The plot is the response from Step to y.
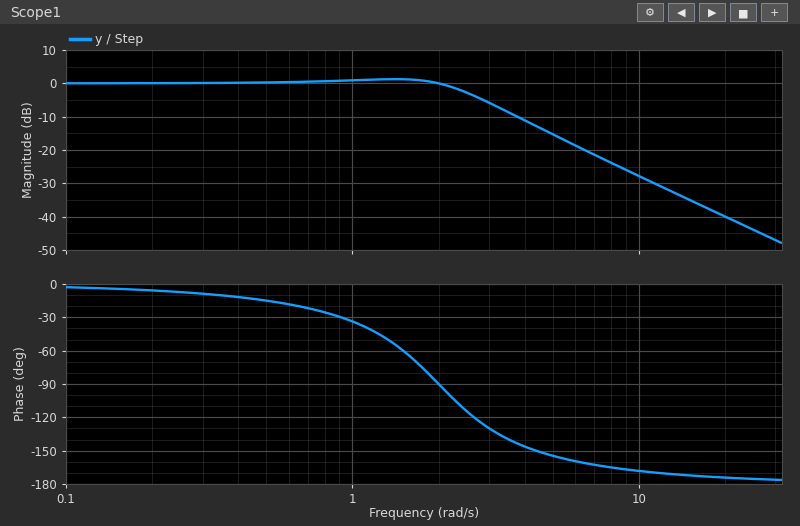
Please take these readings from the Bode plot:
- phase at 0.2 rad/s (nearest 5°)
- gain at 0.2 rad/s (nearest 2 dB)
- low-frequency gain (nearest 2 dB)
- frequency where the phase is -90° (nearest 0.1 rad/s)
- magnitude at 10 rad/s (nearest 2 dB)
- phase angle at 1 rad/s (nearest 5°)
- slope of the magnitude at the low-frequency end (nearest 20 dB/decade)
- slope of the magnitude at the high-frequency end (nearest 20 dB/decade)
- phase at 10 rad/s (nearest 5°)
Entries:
-5°
0 dB
0 dB
2.0 rad/s
-28 dB
-35°
0 dB/decade
-40 dB/decade
-170°
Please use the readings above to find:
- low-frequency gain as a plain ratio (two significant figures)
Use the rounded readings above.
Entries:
1.0
